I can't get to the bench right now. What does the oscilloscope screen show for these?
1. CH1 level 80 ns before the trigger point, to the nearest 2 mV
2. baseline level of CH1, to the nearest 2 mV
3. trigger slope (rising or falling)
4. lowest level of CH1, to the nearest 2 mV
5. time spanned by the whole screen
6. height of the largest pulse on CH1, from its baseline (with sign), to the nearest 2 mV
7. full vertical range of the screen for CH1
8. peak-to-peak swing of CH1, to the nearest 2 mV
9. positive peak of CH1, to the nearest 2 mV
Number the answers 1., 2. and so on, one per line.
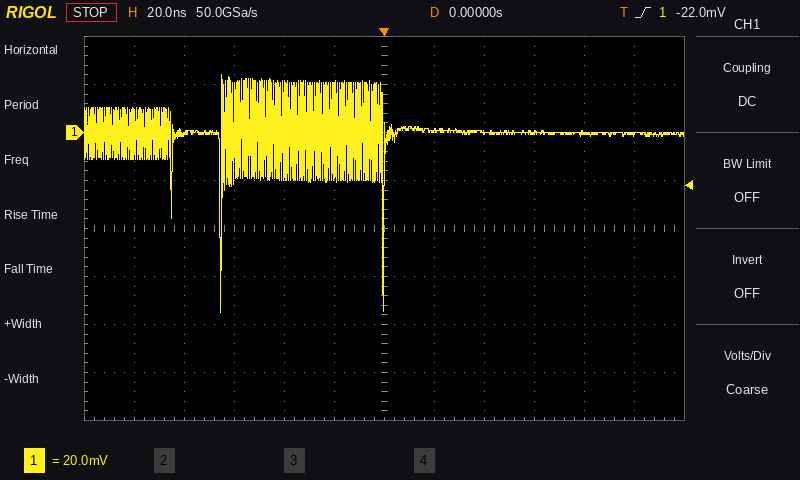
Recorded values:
1. 0 mV
2. 0 mV
3. rising
4. -76 mV
5. 240 ns
6. -76 mV
7. 160 mV
8. 100 mV
9. 24 mV
